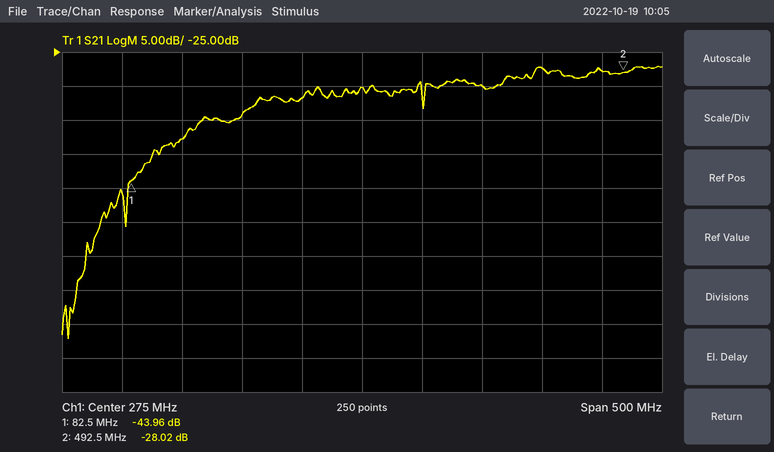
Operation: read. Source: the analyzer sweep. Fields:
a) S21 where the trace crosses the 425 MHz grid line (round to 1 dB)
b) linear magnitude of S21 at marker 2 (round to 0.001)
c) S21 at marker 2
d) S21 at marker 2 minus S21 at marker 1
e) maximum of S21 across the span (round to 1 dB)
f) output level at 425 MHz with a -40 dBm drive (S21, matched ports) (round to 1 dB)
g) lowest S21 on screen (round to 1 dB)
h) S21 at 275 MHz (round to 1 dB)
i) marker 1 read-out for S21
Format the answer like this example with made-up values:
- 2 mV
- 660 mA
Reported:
- -27 dB
- 0.040
- -28.02 dB
- 15.94 dB
- -27 dB
- -67 dBm
- -67 dB
- -30 dB
- -43.96 dB
